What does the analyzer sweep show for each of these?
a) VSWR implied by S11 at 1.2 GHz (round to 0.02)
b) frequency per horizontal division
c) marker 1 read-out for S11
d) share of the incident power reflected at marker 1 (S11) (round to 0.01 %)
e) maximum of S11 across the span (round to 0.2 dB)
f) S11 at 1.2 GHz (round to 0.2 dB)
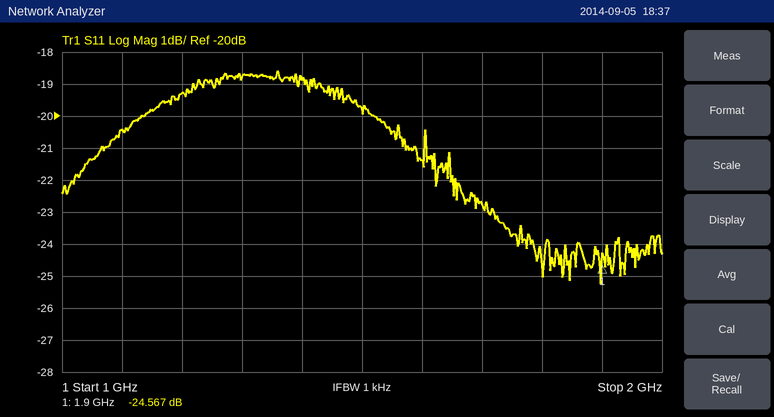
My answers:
1.24
100 MHz
-24.567 dB
0.35 %
-18.6 dB
-19.2 dB
